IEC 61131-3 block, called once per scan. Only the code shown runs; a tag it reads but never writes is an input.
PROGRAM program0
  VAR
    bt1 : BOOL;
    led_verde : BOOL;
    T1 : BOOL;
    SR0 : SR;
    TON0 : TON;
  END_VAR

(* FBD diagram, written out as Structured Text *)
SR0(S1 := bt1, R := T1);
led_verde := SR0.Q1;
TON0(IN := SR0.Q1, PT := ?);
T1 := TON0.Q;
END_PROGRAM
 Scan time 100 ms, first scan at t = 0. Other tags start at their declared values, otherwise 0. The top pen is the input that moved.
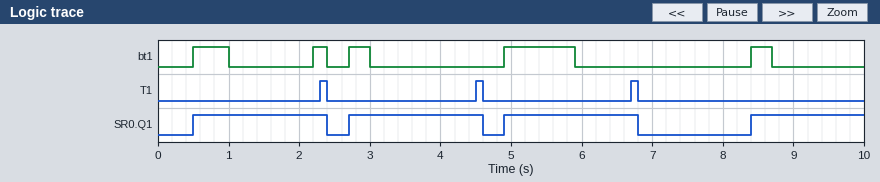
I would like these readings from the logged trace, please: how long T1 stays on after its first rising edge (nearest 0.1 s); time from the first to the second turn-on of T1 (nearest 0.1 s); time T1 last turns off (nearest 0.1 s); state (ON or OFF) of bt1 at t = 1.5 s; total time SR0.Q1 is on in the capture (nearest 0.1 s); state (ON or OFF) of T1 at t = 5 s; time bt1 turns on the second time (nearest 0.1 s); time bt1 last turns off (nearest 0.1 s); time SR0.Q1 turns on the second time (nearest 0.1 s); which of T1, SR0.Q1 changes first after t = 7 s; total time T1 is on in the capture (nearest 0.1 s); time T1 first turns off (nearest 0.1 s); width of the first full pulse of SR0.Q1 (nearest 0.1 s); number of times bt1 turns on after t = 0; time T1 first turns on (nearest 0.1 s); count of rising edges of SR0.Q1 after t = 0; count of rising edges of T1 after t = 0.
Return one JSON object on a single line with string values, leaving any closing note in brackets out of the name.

{"how long T1 stays on after its first rising edge": "0.1 s", "time from the first to the second turn-on of T1": "2.2 s", "time T1 last turns off": "6.8 s", "state (ON or OFF) of bt1 at t = 1.5 s": "OFF", "total time SR0.Q1 is on in the capture": "7.3 s", "state (ON or OFF) of T1 at t = 5 s": "OFF", "time bt1 turns on the second time": "2.2 s", "time bt1 last turns off": "8.7 s", "time SR0.Q1 turns on the second time": "2.7 s", "which of T1, SR0.Q1 changes first after t = 7 s": "SR0.Q1", "total time T1 is on in the capture": "0.3 s", "time T1 first turns off": "2.4 s", "width of the first full pulse of SR0.Q1": "1.9 s", "number of times bt1 turns on after t = 0": "5", "time T1 first turns on": "2.3 s", "count of rising edges of SR0.Q1 after t = 0": "4", "count of rising edges of T1 after t = 0": "3"}
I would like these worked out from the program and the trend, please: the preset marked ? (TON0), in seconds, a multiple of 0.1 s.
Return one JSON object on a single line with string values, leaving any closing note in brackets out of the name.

{"the preset marked ? (TON0), in seconds, a multiple of 0.1 s": "1.8 s"}
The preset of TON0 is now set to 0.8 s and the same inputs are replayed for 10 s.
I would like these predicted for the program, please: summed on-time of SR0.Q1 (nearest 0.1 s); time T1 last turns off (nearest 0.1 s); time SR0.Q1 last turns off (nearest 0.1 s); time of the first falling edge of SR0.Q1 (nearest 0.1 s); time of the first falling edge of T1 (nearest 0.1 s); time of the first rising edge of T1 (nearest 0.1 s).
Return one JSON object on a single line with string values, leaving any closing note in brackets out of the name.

{"summed on-time of SR0.Q1": "3.7 s", "time T1 last turns off": "9.3 s", "time SR0.Q1 last turns off": "9.3 s", "time of the first falling edge of SR0.Q1": "1.4 s", "time of the first falling edge of T1": "1.4 s", "time of the first rising edge of T1": "1.3 s"}
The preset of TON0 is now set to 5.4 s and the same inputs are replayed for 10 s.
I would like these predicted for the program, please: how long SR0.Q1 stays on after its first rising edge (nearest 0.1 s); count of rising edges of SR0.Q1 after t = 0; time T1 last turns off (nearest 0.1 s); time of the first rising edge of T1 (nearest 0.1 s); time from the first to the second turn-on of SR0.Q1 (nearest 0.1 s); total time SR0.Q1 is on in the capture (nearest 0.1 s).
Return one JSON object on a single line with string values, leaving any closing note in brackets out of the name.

{"how long SR0.Q1 stays on after its first rising edge": "5.5 s", "count of rising edges of SR0.Q1 after t = 0": "2", "time T1 last turns off": "6.0 s", "time of the first rising edge of T1": "5.9 s", "time from the first to the second turn-on of SR0.Q1": "7.9 s", "total time SR0.Q1 is on in the capture": "7.1 s"}
